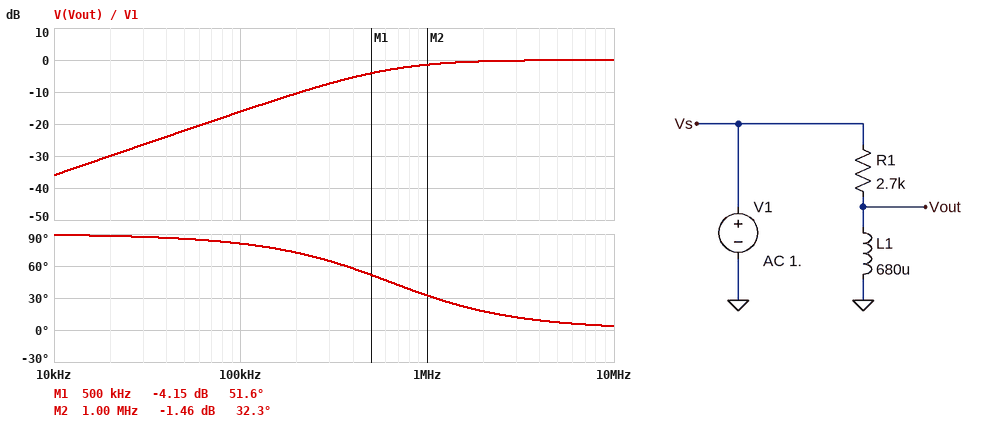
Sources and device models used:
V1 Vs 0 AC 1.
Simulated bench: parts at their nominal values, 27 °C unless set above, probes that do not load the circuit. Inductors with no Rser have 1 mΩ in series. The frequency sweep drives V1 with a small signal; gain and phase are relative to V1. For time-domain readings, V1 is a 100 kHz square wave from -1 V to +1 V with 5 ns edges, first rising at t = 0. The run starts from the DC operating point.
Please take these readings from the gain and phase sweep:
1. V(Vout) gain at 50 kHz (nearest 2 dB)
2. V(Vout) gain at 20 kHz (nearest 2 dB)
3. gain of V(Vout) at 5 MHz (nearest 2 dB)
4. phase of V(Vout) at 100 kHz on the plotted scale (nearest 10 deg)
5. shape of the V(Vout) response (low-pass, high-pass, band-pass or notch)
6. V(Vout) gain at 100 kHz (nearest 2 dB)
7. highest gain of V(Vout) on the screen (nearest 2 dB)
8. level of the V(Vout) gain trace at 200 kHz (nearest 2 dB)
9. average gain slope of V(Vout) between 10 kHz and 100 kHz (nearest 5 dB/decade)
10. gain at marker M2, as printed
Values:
-22 dB
-30 dB
0 dB
80 deg
high-pass
-16 dB
0 dB
-10 dB
20 dB/decade
-1.46 dB
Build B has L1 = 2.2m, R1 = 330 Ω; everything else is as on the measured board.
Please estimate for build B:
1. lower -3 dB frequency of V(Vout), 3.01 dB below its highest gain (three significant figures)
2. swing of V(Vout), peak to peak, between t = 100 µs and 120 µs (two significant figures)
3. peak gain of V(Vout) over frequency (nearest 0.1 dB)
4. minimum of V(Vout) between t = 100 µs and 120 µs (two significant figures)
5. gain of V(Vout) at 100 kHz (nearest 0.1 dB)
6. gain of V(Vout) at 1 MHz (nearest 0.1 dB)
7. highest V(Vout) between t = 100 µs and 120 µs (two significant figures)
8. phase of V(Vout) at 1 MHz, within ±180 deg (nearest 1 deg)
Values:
23.9 kHz
2.7 V
0 dB
-1.4 V
-0.2 dB
0 dB
1.4 V
1 deg
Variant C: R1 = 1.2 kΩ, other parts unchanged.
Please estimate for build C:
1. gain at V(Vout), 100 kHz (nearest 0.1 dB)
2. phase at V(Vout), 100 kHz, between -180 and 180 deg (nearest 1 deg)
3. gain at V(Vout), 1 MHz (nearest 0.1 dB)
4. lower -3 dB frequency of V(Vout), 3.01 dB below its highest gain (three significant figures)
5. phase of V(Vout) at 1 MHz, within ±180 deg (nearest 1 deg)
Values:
-9.5 dB
70 deg
-0.3 dB
281 kHz
16 deg
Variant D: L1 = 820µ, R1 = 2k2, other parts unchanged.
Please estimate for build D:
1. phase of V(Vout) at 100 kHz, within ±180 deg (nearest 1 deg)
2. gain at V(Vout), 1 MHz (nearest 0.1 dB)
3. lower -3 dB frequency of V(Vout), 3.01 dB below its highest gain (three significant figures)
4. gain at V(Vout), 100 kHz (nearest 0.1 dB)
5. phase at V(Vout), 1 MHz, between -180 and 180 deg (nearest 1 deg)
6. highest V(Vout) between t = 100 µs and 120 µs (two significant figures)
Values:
77 deg
-0.7 dB
427 kHz
-12.8 dB
23 deg
2.0 V
